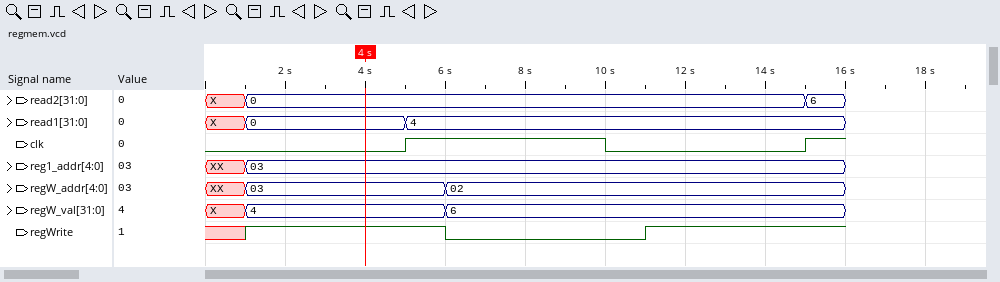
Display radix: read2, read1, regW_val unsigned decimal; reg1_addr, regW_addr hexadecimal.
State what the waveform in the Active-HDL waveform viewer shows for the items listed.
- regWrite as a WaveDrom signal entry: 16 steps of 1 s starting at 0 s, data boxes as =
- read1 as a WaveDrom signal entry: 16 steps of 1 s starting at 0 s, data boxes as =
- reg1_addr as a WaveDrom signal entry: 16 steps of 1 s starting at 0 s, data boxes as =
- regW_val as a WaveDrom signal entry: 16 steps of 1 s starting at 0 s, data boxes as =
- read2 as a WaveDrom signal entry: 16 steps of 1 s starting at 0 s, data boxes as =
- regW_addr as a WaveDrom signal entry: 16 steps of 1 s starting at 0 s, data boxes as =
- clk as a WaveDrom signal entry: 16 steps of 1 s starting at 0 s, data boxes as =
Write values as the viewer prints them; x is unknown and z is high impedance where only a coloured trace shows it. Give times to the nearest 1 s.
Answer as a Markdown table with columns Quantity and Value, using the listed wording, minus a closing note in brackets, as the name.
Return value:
| Quantity | Value |
|---|---|
| regWrite as a WaveDrom signal entry: 16 steps of 1 s starting at 0 s, data boxes as = | {name: 'regWrite', wave: 'x1....0....1....'} |
| read1 as a WaveDrom signal entry: 16 steps of 1 s starting at 0 s, data boxes as = | {name: 'read1', wave: 'x=...=..........', data: '0 4'} |
| reg1_addr as a WaveDrom signal entry: 16 steps of 1 s starting at 0 s, data boxes as = | {name: 'reg1_addr', wave: 'x=..............', data: '03'} |
| regW_val as a WaveDrom signal entry: 16 steps of 1 s starting at 0 s, data boxes as = | {name: 'regW_val', wave: 'x=....=.........', data: '4 6'} |
| read2 as a WaveDrom signal entry: 16 steps of 1 s starting at 0 s, data boxes as = | {name: 'read2', wave: 'x=.............=', data: '0 6'} |
| regW_addr as a WaveDrom signal entry: 16 steps of 1 s starting at 0 s, data boxes as = | {name: 'regW_addr', wave: 'x=....=.........', data: '03 02'} |
| clk as a WaveDrom signal entry: 16 steps of 1 s starting at 0 s, data boxes as = | {name: 'clk', wave: '0....1....0....1'} |
